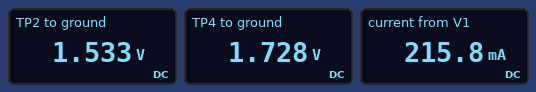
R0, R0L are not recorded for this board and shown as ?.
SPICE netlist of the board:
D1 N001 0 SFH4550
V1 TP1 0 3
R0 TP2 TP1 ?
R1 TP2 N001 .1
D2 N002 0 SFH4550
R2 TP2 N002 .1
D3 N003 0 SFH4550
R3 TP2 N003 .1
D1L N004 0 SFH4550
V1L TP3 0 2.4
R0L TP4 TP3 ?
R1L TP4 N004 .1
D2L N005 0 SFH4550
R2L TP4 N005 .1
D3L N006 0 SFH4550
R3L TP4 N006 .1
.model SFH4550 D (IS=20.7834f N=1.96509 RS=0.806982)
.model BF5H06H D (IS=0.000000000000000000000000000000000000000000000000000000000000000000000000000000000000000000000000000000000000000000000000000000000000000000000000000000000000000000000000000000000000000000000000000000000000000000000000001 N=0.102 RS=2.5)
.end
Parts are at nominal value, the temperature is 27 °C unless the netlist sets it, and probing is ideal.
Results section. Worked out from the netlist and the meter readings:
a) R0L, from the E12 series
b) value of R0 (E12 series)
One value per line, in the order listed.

1 Ω
6.8 Ω
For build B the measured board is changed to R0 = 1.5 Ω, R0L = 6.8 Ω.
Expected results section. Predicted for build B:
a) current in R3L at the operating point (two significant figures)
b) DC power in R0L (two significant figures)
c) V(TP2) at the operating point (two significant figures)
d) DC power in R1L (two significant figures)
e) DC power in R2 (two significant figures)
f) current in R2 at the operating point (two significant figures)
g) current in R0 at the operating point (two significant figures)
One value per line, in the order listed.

45 mA
120 mW
1.8 V
200 µW
7.3 mW
270 mA
810 mA
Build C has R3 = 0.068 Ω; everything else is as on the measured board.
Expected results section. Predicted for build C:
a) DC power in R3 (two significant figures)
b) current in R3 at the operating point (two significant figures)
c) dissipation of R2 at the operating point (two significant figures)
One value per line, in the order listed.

360 µW
73 mA
510 µW
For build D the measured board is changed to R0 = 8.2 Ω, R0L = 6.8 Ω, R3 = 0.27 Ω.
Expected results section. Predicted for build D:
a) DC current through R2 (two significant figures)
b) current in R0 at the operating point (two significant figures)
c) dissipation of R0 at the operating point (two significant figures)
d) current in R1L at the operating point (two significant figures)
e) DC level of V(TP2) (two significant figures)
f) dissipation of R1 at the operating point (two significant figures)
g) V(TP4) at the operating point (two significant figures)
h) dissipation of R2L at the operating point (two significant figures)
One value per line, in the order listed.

62 mA
180 mA
270 mW
45 mA
1.5 V
390 µW
1.5 V
200 µW
